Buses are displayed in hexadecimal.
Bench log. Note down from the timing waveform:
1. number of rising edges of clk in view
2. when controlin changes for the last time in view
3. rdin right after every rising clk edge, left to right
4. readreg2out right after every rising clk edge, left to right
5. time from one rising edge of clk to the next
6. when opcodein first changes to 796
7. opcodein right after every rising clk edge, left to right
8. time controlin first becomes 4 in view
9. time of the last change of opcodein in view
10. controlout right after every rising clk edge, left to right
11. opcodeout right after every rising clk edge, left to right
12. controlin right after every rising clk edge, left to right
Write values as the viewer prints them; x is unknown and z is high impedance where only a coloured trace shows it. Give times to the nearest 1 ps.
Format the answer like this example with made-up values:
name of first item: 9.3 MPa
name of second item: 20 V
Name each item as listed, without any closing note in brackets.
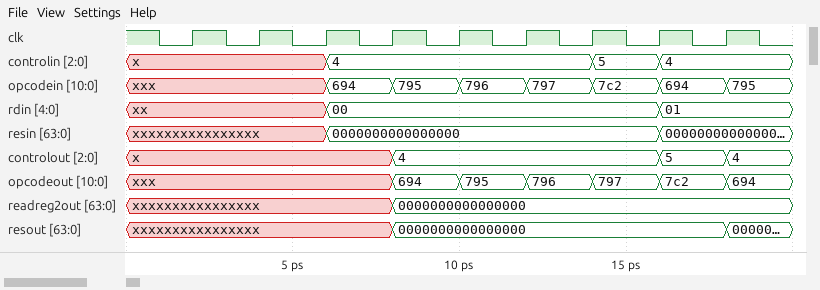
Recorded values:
number of rising edges of clk in view: 9
when controlin changes for the last time in view: 16 ps
rdin right after every rising clk edge, left to right: xx, xx, 00, 00, 00, 00, 00, 01, 01
readreg2out right after every rising clk edge, left to right: xxxxxxxxxxxxxxxx, xxxxxxxxxxxxxxxx, xxxxxxxxxxxxxxxx, 0000000000000000, 0000000000000000, 0000000000000000, 0000000000000000, 0000000000000000, 0000000000000000
time from one rising edge of clk to the next: 2 ps
when opcodein first changes to 796: 10 ps
opcodein right after every rising clk edge, left to right: xxx, xxx, 694, 795, 796, 797, 7c2, 694, 795
time controlin first becomes 4 in view: 6 ps
time of the last change of opcodein in view: 18 ps
controlout right after every rising clk edge, left to right: x, x, x, 4, 4, 4, 4, 5, 4
opcodeout right after every rising clk edge, left to right: xxx, xxx, xxx, 694, 795, 796, 797, 7c2, 694
controlin right after every rising clk edge, left to right: x, x, 4, 4, 4, 4, 5, 4, 4
